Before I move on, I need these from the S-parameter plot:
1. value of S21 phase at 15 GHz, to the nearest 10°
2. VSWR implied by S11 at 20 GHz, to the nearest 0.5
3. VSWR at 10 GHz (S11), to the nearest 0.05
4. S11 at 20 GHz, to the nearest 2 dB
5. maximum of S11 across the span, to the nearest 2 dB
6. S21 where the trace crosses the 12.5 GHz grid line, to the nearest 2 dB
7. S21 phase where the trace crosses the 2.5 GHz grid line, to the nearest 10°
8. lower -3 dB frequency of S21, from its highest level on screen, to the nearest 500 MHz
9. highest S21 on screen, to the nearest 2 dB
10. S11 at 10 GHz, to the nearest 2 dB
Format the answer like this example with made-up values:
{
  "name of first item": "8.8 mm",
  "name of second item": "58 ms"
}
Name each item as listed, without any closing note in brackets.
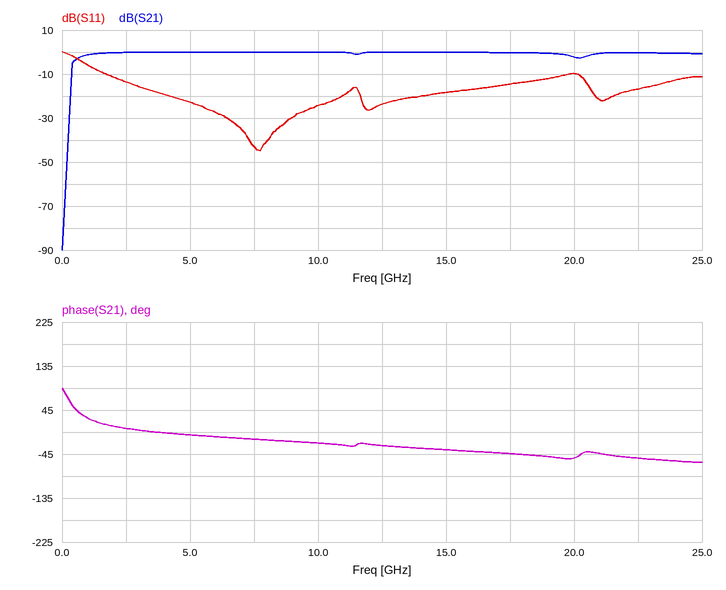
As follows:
{
  "value of S21 phase at 15 GHz, to the nearest 10°": "-40°",
  "VSWR implied by S11 at 20 GHz, to the nearest 0.5": "2.0",
  "VSWR at 10 GHz (S11), to the nearest 0.05": "1.15",
  "S11 at 20 GHz, to the nearest 2 dB": "-10 dB",
  "maximum of S11 across the span, to the nearest 2 dB": "0 dB",
  "S21 where the trace crosses the 12.5 GHz grid line, to the nearest 2 dB": "0 dB",
  "S21 phase where the trace crosses the 2.5 GHz grid line, to the nearest 10°": "10°",
  "lower -3 dB frequency of S21, from its highest level on screen, to the nearest 500 MHz": "500 MHz",
  "highest S21 on screen, to the nearest 2 dB": "0 dB",
  "S11 at 10 GHz, to the nearest 2 dB": "-24 dB"
}
